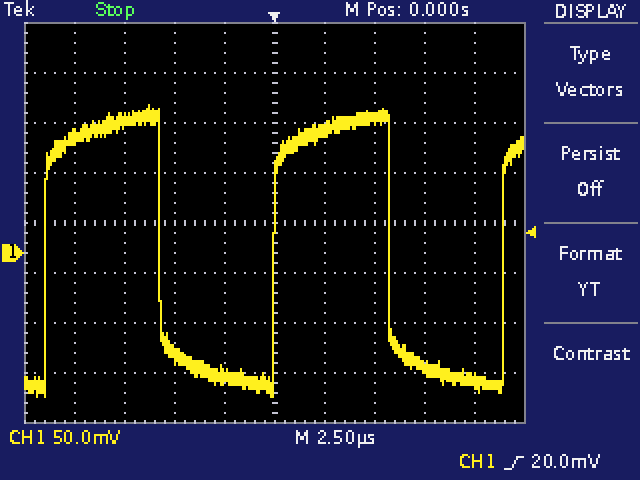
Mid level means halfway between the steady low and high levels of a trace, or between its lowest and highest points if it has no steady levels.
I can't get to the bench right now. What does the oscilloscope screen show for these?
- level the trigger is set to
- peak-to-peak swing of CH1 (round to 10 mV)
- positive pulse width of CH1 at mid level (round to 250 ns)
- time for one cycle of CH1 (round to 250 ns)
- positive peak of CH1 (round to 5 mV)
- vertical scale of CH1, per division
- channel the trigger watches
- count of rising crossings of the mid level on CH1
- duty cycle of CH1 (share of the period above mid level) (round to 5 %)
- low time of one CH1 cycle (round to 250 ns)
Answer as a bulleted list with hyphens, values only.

- 20.0 mV
- 290 mV
- 5.75 µs
- 11.50 µs
- 150 mV
- 50 mV
- CH1
- 3
- 50 %
- 5.75 µs
